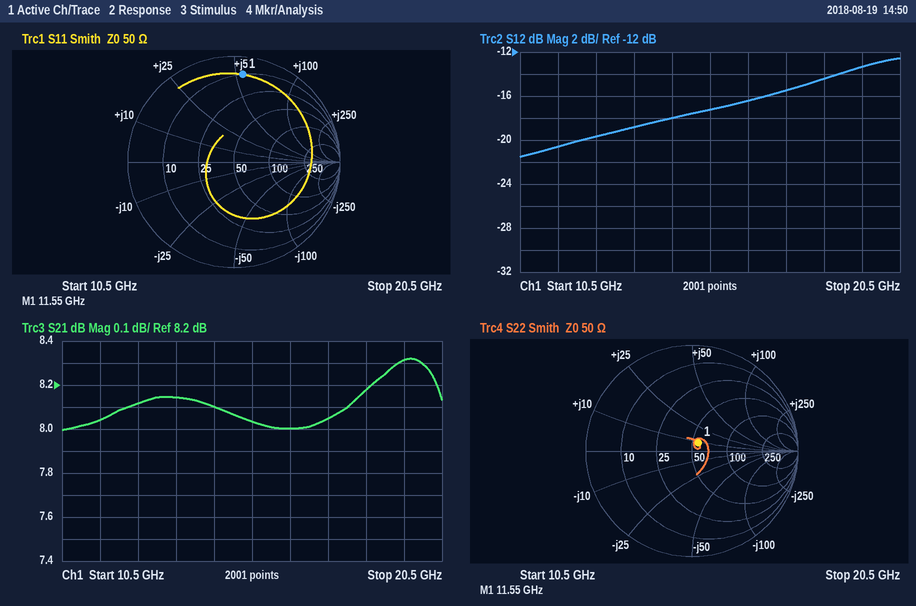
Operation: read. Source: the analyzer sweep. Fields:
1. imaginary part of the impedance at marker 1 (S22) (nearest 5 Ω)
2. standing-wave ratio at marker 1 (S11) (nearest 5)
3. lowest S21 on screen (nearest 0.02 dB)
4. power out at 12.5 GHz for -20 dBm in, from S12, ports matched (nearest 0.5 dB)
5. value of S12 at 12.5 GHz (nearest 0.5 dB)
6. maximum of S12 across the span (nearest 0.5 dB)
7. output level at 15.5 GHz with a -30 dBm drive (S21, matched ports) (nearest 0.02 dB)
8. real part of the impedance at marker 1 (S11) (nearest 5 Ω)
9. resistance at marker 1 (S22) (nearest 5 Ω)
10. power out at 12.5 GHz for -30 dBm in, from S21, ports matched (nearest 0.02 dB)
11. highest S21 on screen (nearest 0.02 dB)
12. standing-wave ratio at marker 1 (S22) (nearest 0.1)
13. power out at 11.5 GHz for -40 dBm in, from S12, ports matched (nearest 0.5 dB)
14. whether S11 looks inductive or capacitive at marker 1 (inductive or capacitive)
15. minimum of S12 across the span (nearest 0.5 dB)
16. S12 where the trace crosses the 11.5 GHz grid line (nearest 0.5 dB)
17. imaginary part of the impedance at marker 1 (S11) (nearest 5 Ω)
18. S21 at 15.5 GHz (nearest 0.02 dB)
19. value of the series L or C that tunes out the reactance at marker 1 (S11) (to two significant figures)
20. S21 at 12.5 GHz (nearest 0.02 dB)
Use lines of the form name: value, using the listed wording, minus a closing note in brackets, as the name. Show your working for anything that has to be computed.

imaginary part of the impedance at marker 1 (S22): +10 Ω
standing-wave ratio at marker 1 (S11): 10
lowest S21 on screen: 8.00 dB
power out at 12.5 GHz for -20 dBm in, from S12, ports matched: -20 dBm + (-19.5 dB) = -39.5 dBm
value of S12 at 12.5 GHz: -19.5 dB
maximum of S12 across the span: -12.5 dB
output level at 15.5 GHz with a -30 dBm drive (S21, matched ports): -30 dBm + (8.04 dB) = -21.96 dBm
real part of the impedance at marker 1 (S11): 10 Ω
resistance at marker 1 (S22): 55 Ω
power out at 12.5 GHz for -30 dBm in, from S21, ports matched: -30 dBm + (8.12 dB) = -21.88 dBm
highest S21 on screen: 8.32 dB
standing-wave ratio at marker 1 (S22): 1.2
power out at 11.5 GHz for -40 dBm in, from S12, ports matched: -40 dBm + (-20.5 dB) = -60.5 dBm
whether S11 looks inductive or capacitive at marker 1: inductive
minimum of S12 across the span: -21.5 dB
S12 where the trace crosses the 11.5 GHz grid line: -20.5 dB
imaginary part of the impedance at marker 1 (S11): +55 Ω
S21 at 15.5 GHz: 8.04 dB
value of the series L or C that tunes out the reactance at marker 1 (S11): C = 1/(2π × 11.55 GHz × 55 Ω) ≈ 251 fF, so 250 fF to two significant figures
S21 at 12.5 GHz: 8.12 dB
